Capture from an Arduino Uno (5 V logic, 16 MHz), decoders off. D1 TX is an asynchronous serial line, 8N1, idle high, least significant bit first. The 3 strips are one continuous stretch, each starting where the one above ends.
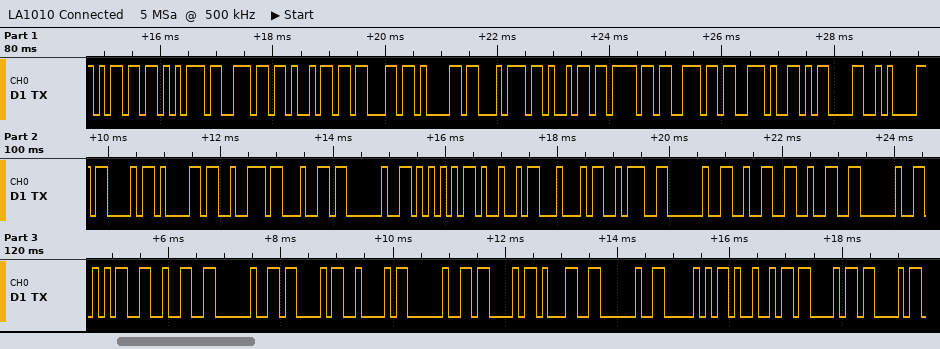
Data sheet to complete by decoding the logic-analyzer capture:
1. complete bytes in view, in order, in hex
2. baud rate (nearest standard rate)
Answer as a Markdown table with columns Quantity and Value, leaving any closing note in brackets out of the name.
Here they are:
| Quantity | Value |
|---|---|
| complete bytes in view, in order, in hex | 6D 75 6E 69 63 61 74 69 6F 6E 2E 0D 0A 43 61 72 64 20 55 49 44 3A 20 32 32 20 35 32 20 43 42 20 43 31 20 50 49 43 43 |
| baud rate | 9600 baud |
